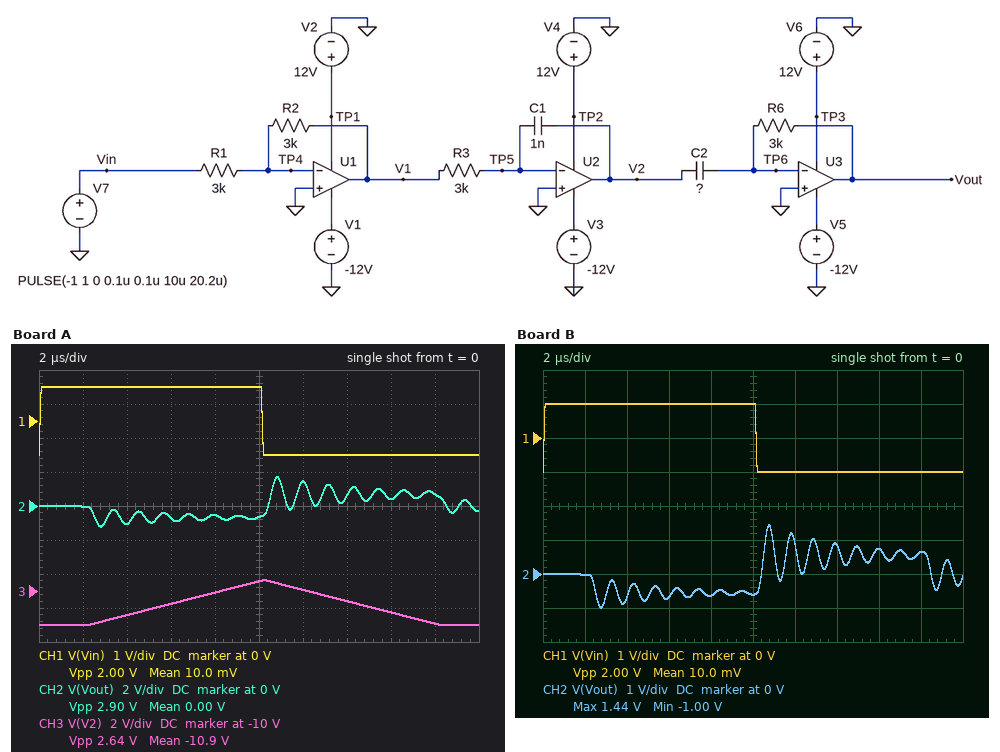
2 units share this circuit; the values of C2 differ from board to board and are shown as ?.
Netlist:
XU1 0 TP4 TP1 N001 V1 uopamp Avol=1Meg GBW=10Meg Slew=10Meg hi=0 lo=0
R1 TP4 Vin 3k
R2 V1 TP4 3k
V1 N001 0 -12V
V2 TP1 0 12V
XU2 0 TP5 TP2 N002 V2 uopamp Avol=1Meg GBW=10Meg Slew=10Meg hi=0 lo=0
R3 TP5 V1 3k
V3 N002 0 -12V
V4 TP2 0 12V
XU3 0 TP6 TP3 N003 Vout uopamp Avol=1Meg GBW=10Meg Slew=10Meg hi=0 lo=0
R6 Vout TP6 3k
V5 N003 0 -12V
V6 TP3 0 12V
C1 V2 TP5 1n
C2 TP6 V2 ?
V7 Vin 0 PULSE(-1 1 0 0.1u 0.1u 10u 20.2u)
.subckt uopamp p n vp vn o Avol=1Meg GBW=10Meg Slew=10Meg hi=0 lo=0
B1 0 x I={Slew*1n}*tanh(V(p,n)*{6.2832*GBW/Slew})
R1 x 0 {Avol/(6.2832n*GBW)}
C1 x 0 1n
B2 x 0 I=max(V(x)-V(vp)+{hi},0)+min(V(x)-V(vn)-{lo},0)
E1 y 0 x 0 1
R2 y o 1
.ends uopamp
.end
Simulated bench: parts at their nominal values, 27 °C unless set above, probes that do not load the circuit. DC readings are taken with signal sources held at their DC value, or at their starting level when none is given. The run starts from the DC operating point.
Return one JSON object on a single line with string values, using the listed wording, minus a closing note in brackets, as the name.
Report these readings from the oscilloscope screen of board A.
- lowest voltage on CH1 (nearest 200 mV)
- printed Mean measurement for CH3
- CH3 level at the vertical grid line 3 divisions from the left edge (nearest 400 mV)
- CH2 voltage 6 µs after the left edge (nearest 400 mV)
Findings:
{"lowest voltage on CH1": "-1.0 V", "printed Mean measurement for CH3": "-10.9 V", "CH3 level at the vertical grid line 3 divisions from the left edge": "-10.8 V", "CH2 voltage 6 µs after the left edge": "-800 mV"}
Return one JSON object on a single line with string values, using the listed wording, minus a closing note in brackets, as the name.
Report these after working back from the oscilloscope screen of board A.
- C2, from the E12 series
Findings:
{"C2, from the E12 series": "680 pF"}
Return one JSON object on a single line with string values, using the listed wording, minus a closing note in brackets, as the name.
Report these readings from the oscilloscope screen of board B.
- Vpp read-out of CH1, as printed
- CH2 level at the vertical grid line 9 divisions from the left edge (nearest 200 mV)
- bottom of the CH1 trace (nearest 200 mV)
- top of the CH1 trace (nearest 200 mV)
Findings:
{"Vpp read-out of CH1, as printed": "2.00 V", "CH2 level at the vertical grid line 9 divisions from the left edge": "600 mV", "bottom of the CH1 trace": "-1.0 V", "top of the CH1 trace": "1.0 V"}
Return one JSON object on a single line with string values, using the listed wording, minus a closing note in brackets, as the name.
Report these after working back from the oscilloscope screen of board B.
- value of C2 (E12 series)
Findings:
{"value of C2": "560 pF"}
